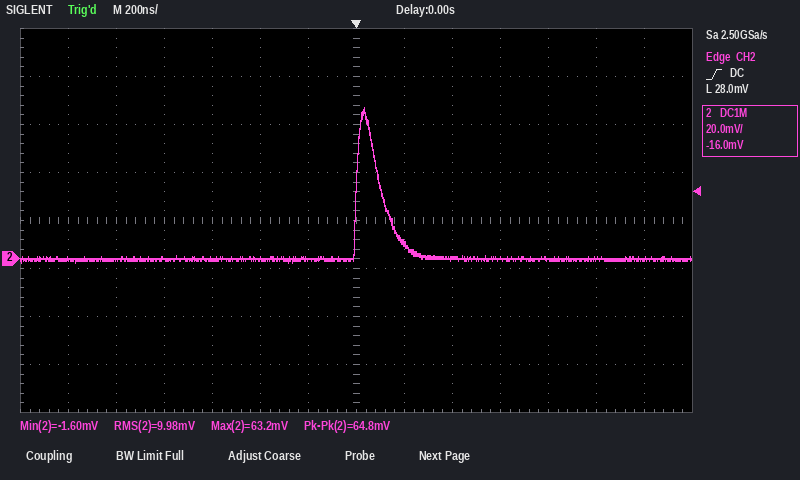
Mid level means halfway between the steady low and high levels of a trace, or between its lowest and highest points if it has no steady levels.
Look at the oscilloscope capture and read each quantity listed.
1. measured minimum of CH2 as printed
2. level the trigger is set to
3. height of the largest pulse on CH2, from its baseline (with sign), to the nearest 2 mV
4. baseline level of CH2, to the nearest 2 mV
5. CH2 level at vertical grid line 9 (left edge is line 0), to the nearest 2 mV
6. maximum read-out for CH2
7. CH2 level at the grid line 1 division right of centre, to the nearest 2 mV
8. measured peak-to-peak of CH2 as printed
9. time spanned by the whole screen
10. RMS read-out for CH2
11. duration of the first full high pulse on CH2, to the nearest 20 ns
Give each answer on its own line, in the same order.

-1.60 mV
28.0 mV
+64 mV
0 mV
0 mV
63.2 mV
6 mV
64.8 mV
2.8 µs
9.98 mV
100 ns
